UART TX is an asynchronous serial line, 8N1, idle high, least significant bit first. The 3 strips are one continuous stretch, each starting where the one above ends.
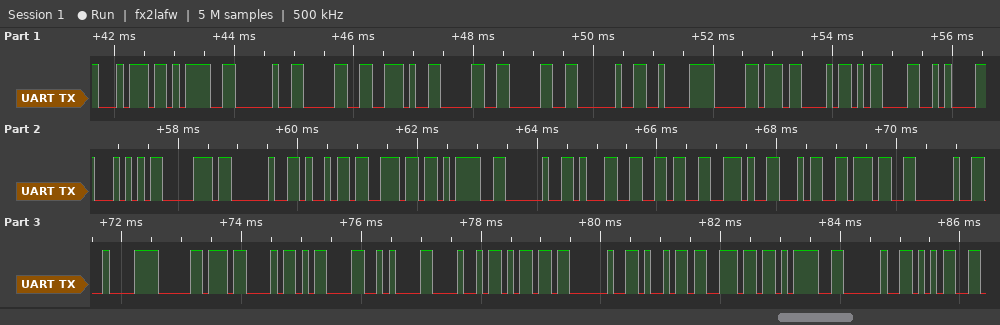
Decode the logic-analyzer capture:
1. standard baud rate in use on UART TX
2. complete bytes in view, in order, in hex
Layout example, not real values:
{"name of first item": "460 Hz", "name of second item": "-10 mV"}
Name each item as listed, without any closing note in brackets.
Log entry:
{"standard baud rate in use on UART TX": "9600 baud", "complete bytes in view, in order, in hex": "74 3D 20 30 2E 30 30 20 C2 B0 43 0D 0A 54 70 20 69 6E 3D 20 31 36 2E 34 37 20 C2 B0 43 0D 0A 48 6D 20 69 6E 3D 20 35"}
